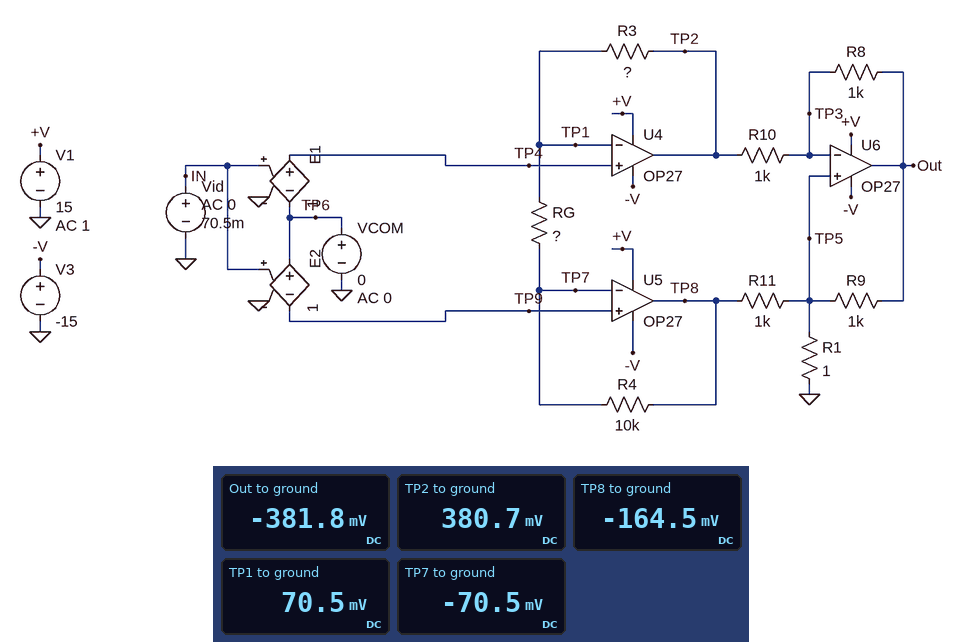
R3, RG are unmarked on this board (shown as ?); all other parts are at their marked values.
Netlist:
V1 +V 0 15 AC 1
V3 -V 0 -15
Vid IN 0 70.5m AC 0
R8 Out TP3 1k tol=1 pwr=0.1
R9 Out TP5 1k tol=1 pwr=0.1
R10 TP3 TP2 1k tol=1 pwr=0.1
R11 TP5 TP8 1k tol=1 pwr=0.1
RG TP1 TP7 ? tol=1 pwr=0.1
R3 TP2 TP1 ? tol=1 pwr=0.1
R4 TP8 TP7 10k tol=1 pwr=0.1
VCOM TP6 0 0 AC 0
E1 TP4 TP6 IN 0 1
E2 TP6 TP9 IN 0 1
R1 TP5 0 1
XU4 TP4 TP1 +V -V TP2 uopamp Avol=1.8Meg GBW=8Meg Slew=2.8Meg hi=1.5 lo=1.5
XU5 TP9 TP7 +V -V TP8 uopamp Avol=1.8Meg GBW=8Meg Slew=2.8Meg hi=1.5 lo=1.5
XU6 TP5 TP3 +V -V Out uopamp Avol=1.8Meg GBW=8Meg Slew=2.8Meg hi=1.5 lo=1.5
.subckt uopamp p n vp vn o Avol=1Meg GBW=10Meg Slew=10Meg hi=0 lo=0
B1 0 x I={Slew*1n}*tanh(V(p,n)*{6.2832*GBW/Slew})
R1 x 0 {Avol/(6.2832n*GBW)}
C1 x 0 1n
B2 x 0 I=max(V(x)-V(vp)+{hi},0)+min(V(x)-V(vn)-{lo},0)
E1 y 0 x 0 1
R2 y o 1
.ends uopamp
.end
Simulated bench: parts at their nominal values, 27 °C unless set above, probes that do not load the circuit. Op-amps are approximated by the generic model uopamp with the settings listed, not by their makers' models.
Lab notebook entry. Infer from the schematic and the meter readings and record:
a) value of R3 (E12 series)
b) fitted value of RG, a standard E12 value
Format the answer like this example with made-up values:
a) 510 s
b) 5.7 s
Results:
a) 33 kΩ
b) 15 kΩ
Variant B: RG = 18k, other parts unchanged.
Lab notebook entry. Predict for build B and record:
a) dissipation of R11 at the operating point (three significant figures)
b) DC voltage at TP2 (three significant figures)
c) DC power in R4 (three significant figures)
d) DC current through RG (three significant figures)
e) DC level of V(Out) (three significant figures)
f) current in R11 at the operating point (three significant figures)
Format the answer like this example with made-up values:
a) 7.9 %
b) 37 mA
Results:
a) 22.0 µW
b) 329 mV
c) 614 nW
d) 7.83 µA
e) -330 mV
f) 148 µA
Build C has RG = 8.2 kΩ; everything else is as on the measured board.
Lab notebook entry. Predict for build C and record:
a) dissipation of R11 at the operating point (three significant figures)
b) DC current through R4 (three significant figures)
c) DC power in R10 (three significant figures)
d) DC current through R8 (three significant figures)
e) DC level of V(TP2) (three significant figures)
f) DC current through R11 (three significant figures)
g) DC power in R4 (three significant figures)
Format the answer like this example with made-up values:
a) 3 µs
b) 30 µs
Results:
a) 58.4 µW
b) 17.2 µA
c) 408 µW
d) 639 µA
e) 638 mV
f) 242 µA
g) 2.96 µW
